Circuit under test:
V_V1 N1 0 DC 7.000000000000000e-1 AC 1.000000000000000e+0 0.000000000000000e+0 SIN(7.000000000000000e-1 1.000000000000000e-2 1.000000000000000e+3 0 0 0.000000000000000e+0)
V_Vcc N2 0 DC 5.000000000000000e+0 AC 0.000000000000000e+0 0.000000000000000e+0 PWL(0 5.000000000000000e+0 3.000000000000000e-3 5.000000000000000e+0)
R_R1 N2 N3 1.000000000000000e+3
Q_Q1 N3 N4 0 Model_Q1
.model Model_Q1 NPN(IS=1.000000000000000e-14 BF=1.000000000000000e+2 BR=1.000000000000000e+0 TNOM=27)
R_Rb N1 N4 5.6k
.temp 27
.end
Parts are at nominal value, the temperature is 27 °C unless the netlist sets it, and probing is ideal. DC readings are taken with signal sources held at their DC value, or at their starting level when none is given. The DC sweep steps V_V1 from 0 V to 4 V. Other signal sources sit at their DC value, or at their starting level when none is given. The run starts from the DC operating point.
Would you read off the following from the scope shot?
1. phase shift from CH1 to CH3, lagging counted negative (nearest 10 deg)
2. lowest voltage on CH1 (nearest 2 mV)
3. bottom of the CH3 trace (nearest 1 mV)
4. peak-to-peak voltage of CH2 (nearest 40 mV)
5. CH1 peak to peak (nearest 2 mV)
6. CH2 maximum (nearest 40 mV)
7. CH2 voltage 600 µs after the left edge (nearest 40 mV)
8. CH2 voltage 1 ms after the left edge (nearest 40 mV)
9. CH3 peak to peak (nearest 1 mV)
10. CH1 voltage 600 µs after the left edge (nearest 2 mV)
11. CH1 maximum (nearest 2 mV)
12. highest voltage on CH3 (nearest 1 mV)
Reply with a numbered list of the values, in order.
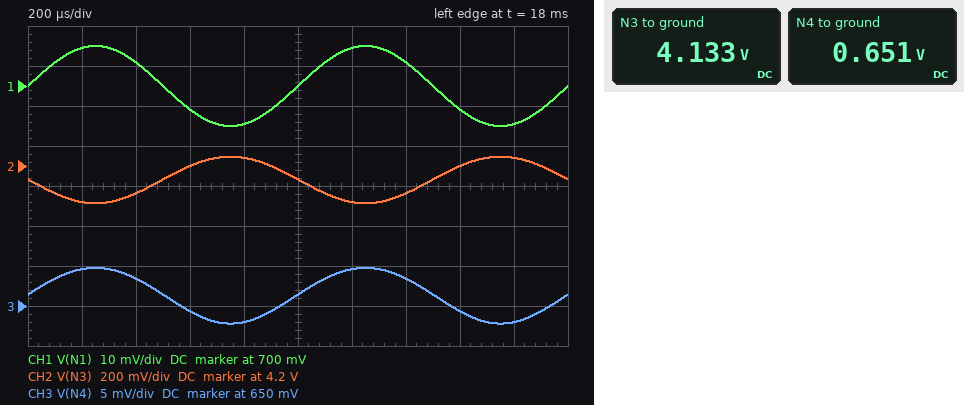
1. 0 deg
2. 690 mV
3. 648 mV
4. 240 mV
5. 20 mV
6. 4.24 V
7. 4.20 V
8. 4.12 V
9. 7 mV
10. 694 mV
11. 710 mV
12. 655 mV
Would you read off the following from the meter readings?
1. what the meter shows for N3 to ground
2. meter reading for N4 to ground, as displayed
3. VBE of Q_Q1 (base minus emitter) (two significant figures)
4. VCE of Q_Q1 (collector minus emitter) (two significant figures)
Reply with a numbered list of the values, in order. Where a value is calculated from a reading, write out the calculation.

1. 4.133 V
2. 0.651 V
3. 651 mV = 650 mV
4. 4.133 V = 4.1 V
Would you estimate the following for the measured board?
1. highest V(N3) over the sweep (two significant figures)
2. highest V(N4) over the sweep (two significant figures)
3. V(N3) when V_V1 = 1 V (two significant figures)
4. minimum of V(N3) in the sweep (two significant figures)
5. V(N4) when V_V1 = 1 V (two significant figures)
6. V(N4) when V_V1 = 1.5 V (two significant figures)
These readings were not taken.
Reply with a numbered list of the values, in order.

1. 5.0 V
2. 700 mV
3. 170 mV
4. 63 mV
5. 700 mV
6. 700 mV
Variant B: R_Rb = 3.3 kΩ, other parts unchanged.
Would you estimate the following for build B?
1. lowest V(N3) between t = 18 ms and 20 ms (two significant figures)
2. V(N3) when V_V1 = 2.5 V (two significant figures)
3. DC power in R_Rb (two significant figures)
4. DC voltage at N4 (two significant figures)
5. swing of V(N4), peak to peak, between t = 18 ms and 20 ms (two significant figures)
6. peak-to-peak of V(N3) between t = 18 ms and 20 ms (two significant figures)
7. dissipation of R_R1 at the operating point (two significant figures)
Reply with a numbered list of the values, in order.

1. 3.6 V
2. 65 mV
3. 480 nW
4. 660 mV
5. 7.9 mV
6. 370 mV
7. 1.5 mW
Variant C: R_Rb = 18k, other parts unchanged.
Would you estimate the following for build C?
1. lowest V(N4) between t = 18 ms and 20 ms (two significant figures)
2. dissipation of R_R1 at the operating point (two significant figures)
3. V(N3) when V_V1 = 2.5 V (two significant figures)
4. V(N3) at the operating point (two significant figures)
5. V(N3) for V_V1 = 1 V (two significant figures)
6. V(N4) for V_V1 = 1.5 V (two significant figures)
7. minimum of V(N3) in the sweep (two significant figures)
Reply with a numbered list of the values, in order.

1. 630 mV
2. 150 µW
3. 120 mV
4. 4.6 V
5. 3.2 V
6. 690 mV
7. 95 mV
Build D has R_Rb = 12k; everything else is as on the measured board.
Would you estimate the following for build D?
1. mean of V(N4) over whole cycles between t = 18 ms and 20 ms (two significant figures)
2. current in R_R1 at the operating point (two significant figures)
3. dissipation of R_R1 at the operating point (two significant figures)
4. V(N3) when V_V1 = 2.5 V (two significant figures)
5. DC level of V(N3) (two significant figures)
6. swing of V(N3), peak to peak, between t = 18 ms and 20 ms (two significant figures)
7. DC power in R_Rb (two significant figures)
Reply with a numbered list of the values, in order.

1. 640 mV
2. 520 µA
3. 270 µW
4. 100 mV
5. 4.5 V
6. 120 mV
7. 320 nW
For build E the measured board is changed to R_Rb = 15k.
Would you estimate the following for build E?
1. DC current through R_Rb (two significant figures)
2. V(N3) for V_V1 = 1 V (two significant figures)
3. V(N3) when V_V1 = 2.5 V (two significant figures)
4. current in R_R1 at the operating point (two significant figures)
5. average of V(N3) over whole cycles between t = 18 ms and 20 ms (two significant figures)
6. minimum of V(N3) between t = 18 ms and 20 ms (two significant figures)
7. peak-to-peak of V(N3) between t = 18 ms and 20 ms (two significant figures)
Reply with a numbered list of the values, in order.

1. 4.4 µA
2. 2.8 V
3. 110 mV
4. 440 µA
5. 4.6 V
6. 4.5 V
7. 96 mV
